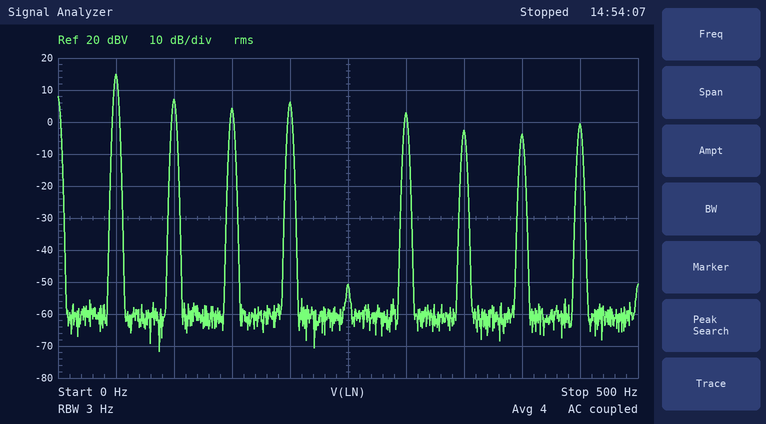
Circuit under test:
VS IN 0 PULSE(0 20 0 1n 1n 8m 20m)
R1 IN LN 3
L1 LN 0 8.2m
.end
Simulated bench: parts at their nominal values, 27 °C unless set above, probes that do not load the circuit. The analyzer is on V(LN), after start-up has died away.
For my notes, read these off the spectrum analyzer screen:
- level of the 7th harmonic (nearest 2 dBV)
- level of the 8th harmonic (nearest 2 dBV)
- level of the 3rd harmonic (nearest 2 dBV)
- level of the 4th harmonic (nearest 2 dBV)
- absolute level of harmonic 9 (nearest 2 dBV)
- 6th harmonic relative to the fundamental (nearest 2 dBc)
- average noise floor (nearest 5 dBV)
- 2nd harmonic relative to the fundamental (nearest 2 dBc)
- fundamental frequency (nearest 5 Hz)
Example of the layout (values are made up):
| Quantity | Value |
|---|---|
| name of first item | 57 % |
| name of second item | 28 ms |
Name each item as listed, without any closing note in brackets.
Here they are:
| Quantity | Value |
|---|---|
| level of the 7th harmonic | -2 dBV |
| level of the 8th harmonic | -4 dBV |
| level of the 3rd harmonic | 4 dBV |
| level of the 4th harmonic | 6 dBV |
| absolute level of harmonic 9 | 0 dBV |
| 6th harmonic relative to the fundamental | -12 dBc |
| average noise floor | -60 dBV |
| 2nd harmonic relative to the fundamental | -8 dBc |
| fundamental frequency | 50 Hz |
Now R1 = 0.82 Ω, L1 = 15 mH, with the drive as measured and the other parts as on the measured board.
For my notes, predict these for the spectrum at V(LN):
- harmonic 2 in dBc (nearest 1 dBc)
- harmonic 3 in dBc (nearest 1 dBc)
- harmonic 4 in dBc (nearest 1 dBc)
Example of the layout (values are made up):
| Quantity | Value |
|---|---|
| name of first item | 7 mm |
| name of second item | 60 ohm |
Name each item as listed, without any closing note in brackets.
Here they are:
| Quantity | Value |
|---|---|
| harmonic 2 in dBc | -10 dBc |
| harmonic 3 in dBc | -14 dBc |
| harmonic 4 in dBc | -12 dBc |
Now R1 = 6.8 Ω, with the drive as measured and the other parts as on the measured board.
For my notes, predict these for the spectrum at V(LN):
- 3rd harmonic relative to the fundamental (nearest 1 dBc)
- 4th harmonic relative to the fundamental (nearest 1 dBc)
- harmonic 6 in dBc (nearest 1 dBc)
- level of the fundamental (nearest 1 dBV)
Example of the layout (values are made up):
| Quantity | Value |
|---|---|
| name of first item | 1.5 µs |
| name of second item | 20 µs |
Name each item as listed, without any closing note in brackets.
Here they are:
| Quantity | Value |
|---|---|
| 3rd harmonic relative to the fundamental | -7 dBc |
| 4th harmonic relative to the fundamental | -5 dBc |
| harmonic 6 in dBc | -7 dBc |
| level of the fundamental | 10 dBV |
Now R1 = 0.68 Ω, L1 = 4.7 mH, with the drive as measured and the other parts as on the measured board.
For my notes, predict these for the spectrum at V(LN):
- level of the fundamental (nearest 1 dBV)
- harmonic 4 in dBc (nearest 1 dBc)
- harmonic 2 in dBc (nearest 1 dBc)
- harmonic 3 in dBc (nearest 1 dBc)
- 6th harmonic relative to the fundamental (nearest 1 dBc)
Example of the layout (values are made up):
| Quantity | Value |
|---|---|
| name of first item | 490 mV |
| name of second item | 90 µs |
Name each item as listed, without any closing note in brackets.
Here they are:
| Quantity | Value |
|---|---|
| level of the fundamental | 18 dBV |
| harmonic 4 in dBc | -11 dBc |
| harmonic 2 in dBc | -10 dBc |
| harmonic 3 in dBc | -13 dBc |
| 6th harmonic relative to the fundamental | -15 dBc |
